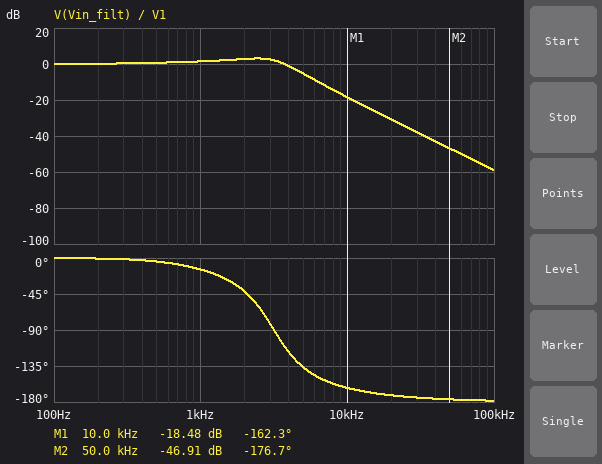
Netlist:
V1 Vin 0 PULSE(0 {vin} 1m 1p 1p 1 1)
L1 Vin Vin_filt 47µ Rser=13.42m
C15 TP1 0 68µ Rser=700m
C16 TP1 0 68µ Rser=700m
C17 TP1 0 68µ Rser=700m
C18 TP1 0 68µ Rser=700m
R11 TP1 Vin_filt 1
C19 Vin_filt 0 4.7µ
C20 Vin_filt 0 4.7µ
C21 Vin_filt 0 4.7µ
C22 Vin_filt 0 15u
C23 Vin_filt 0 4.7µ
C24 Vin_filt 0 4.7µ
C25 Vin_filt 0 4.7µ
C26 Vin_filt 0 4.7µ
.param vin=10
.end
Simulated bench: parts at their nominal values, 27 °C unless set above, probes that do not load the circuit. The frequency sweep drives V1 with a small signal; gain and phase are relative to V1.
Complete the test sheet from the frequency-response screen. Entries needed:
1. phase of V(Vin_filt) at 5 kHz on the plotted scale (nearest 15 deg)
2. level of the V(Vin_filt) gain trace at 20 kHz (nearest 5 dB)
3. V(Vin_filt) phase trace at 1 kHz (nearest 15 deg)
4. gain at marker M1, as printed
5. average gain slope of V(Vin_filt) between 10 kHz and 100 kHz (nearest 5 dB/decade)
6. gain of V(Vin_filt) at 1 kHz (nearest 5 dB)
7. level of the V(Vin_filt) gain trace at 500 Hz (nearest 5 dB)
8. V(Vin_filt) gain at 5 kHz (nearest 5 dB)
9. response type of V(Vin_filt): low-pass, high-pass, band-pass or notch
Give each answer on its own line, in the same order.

-135 deg
-30 dB
-15 deg
-18.48 dB
-40 dB/decade
0 dB
0 dB
-5 dB
low-pass
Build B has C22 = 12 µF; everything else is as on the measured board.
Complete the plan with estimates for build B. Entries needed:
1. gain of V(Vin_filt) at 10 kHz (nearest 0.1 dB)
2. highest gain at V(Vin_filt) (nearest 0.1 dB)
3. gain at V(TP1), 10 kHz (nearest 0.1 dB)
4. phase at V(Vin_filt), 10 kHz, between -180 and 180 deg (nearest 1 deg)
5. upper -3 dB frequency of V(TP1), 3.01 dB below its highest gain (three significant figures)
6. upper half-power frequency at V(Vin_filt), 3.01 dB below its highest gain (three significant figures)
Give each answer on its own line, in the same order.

-17.9 dB
2.9 dB
-34.0 dB
-161 deg
614 Hz
3.82 kHz
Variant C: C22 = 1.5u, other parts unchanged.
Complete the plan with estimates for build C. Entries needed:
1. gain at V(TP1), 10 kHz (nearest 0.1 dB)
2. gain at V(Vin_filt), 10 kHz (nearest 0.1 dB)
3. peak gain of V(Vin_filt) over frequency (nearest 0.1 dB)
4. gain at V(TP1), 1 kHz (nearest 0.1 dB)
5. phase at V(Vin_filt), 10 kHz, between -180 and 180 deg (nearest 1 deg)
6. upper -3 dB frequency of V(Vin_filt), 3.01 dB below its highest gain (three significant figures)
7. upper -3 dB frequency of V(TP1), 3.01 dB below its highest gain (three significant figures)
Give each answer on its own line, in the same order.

-31.7 dB
-15.6 dB
2.1 dB
-5.4 dB
-155 deg
4.28 kHz
604 Hz
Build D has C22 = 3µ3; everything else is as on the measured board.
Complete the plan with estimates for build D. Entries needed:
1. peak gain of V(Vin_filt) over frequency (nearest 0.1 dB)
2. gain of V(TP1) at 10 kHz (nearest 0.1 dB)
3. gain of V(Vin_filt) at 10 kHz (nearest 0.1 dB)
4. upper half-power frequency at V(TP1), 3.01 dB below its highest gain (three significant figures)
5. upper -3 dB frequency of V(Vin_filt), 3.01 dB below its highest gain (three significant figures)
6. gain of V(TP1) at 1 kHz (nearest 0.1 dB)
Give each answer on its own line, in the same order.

2.2 dB
-32.2 dB
-16.1 dB
606 Hz
4.20 kHz
-5.4 dB
